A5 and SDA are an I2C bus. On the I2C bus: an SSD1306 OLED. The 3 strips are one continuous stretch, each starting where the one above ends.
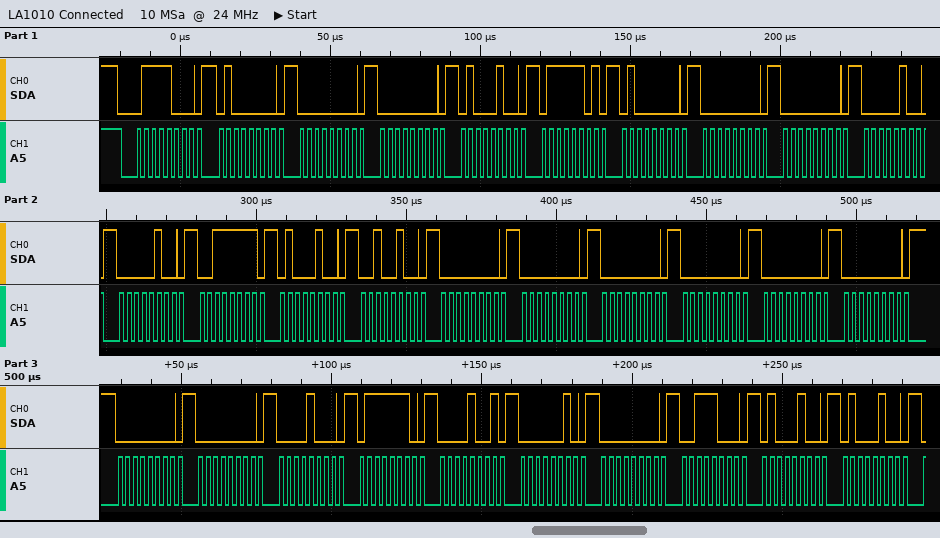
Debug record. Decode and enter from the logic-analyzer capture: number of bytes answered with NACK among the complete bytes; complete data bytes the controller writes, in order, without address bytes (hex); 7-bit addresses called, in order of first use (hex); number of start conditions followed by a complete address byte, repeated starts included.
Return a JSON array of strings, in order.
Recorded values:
["0", "40 00 00 44 7D 40 00 00 04 04 3F 44 24 00 00 00 00 00 00 00 00 08 7E 09 02 00 38 44 44", "0x3C", "1"]
